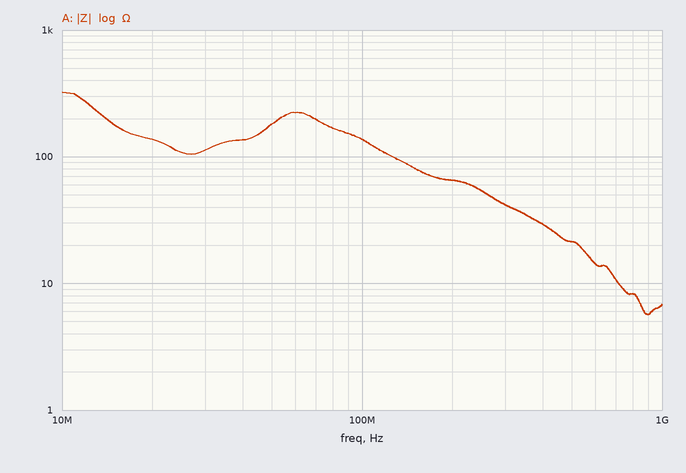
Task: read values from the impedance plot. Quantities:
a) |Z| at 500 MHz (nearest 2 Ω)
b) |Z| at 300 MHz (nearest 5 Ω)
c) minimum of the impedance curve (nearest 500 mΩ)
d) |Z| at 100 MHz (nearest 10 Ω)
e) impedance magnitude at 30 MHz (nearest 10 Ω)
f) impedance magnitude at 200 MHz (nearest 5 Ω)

22 Ω
40 Ω
5.5 Ω
140 Ω
110 Ω
65 Ω
